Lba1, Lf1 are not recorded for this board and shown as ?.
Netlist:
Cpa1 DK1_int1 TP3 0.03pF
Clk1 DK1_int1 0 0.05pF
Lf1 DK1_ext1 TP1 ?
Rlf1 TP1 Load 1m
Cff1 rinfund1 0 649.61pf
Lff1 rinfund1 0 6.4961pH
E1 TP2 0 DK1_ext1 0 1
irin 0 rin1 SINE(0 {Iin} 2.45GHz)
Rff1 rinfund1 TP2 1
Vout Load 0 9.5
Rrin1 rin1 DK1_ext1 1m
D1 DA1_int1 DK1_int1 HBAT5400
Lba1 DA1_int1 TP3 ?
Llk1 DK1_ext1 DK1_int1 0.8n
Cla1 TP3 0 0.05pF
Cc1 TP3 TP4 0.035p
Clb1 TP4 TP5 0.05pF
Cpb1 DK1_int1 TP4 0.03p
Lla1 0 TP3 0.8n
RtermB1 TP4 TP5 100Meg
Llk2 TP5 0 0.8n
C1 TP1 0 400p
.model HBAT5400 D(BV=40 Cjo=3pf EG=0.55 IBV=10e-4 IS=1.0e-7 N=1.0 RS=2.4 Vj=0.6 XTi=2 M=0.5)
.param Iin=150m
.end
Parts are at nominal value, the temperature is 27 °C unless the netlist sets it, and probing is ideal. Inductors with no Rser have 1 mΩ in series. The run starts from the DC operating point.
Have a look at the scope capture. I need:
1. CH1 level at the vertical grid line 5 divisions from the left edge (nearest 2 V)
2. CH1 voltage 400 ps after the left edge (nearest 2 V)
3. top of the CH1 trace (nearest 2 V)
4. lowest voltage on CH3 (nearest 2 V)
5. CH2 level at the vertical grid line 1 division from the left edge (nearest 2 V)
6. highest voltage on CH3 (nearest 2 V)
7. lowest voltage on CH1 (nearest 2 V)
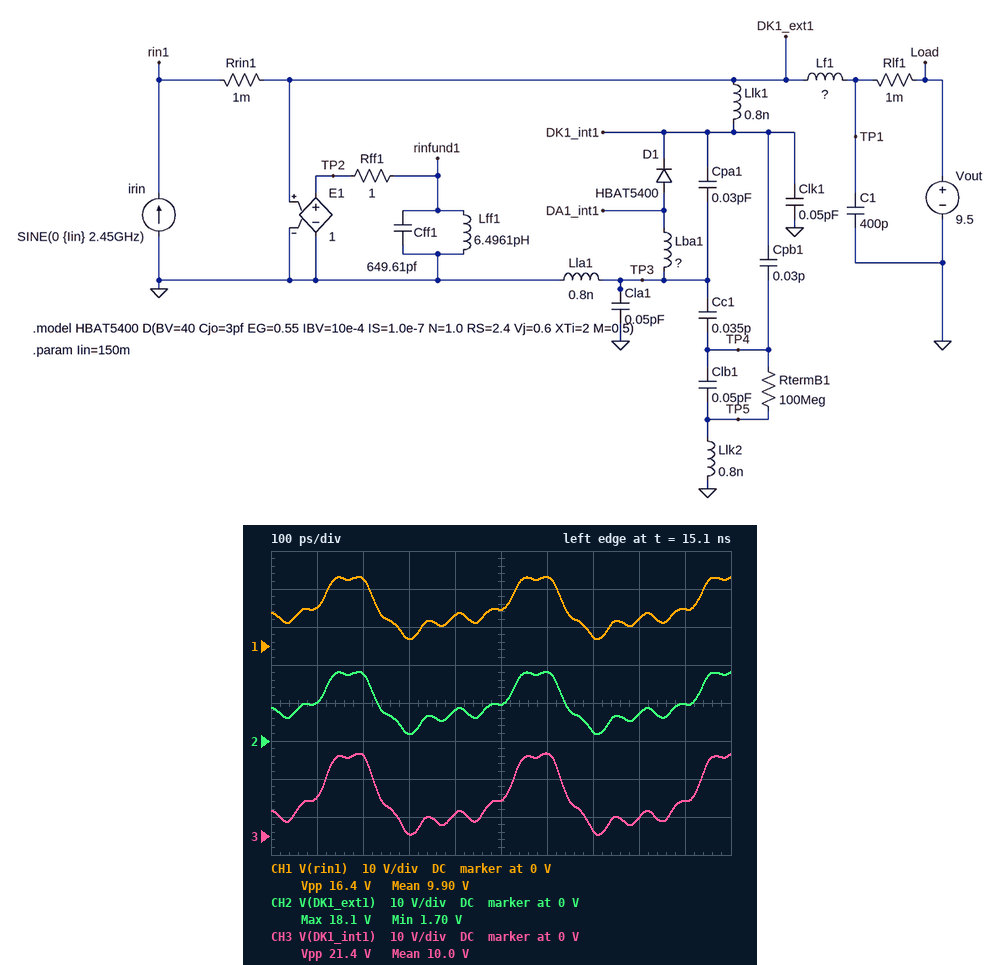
10 V
8 V
18 V
0 V
10 V
22 V
2 V
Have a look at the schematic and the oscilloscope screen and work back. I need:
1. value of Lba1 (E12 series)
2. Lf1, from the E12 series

1 nH
3.9 nH
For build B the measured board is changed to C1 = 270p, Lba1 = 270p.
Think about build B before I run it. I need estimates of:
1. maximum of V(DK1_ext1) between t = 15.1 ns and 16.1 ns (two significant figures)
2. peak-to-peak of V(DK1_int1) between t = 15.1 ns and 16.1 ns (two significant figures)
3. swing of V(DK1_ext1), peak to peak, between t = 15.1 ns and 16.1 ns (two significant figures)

22 V
26 V
21 V
